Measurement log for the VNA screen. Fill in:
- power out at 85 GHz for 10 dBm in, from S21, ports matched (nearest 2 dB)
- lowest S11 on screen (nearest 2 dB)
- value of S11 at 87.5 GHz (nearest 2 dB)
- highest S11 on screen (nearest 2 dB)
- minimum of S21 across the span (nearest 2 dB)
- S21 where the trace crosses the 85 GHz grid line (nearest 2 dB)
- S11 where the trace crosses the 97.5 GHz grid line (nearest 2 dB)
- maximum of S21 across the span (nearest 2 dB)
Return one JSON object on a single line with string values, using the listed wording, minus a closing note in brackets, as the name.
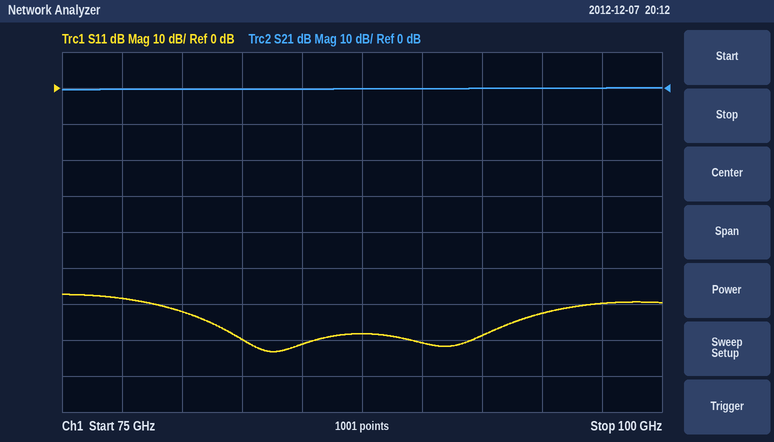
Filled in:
{"power out at 85 GHz for 10 dBm in, from S21, ports matched": "10 dBm", "lowest S11 on screen": "-74 dB", "value of S11 at 87.5 GHz": "-68 dB", "highest S11 on screen": "-58 dB", "minimum of S21 across the span": "0 dB", "S21 where the trace crosses the 85 GHz grid line": "0 dB", "S11 where the trace crosses the 97.5 GHz grid line": "-60 dB", "maximum of S21 across the span": "0 dB"}
